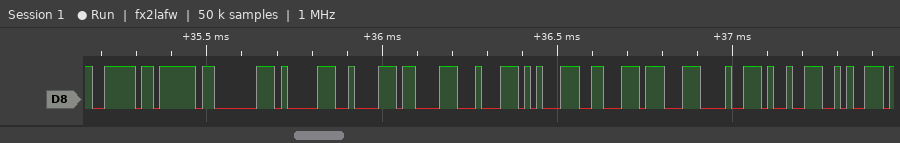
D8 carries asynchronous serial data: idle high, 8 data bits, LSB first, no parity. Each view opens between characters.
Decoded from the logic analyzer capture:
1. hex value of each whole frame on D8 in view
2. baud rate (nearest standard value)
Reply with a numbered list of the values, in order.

1. BE, BF, C0, C1, C2, C3, C4, C5, C6, C7, C8, C9, CA
2. 57600 baud
